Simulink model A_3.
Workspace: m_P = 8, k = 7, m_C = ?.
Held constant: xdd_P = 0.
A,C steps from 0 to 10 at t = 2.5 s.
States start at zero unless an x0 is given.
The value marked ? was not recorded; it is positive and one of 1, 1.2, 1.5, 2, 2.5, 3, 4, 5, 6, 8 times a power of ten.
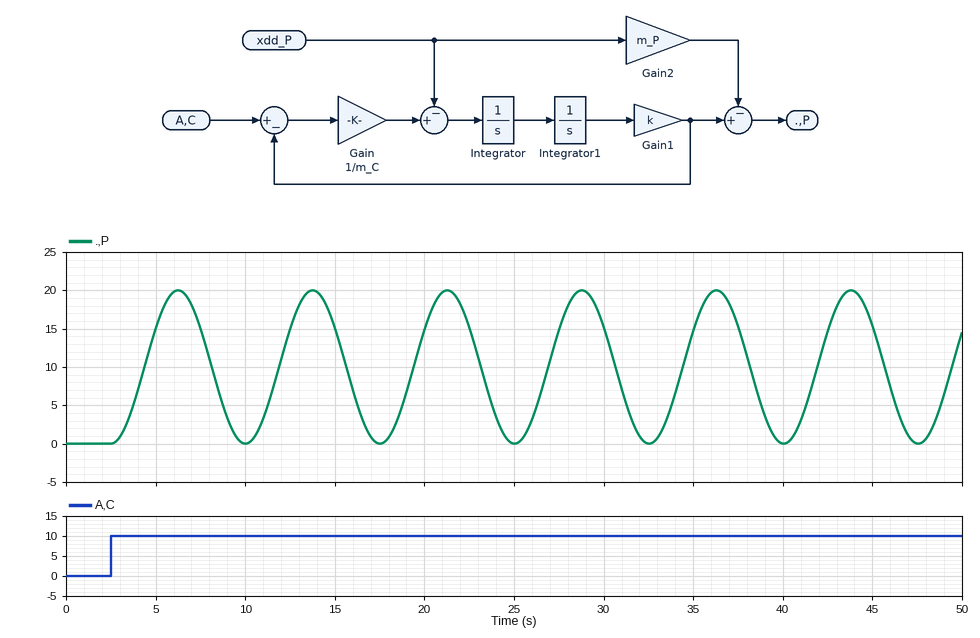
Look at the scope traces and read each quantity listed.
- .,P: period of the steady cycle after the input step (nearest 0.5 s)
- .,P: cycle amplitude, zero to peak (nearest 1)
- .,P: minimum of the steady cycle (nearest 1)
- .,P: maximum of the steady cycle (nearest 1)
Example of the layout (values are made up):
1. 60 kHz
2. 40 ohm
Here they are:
1. 7.5 s
2. 10
3. 0
4. 20
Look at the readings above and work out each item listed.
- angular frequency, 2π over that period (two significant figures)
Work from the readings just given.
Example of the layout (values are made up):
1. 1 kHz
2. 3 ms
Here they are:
1. 0.84 rad/s
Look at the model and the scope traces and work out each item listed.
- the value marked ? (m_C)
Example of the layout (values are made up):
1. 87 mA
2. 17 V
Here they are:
1. 10
